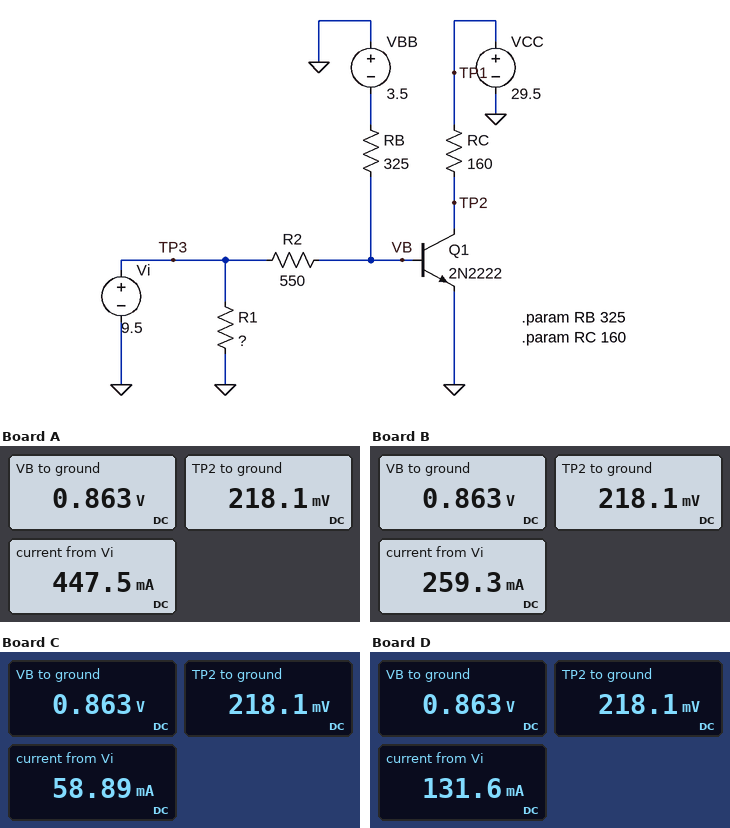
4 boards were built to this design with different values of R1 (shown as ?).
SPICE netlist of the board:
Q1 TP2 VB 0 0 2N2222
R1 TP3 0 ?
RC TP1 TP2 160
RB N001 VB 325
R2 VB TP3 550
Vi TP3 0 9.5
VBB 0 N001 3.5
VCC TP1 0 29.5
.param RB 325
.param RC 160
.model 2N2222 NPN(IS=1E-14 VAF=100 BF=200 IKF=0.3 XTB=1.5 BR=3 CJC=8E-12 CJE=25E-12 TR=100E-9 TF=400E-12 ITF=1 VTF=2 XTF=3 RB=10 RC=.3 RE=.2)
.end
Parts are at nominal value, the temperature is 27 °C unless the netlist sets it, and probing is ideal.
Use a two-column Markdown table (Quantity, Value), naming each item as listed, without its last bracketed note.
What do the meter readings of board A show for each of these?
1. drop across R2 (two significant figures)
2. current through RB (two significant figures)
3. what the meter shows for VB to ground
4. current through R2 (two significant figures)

| Quantity | Value |
|---|---|
| drop across R2 | 8.6 V |
| current through RB | 13 mA |
| what the meter shows for VB to ground | 0.863 V |
| current through R2 | 16 mA |
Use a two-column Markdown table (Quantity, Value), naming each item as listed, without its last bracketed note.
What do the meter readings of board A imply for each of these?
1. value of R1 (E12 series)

| Quantity | Value |
|---|---|
| value of R1 | 22 Ω |
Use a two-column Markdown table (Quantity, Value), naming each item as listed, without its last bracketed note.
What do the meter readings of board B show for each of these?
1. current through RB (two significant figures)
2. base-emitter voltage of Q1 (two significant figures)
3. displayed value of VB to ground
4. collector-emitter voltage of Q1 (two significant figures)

| Quantity | Value |
|---|---|
| current through RB | 13 mA |
| base-emitter voltage of Q1 | 860 mV |
| displayed value of VB to ground | 0.863 V |
| collector-emitter voltage of Q1 | 220 mV |
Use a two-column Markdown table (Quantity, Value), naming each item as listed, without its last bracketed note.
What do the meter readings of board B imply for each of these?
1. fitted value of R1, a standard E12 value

| Quantity | Value |
|---|---|
| fitted value of R1, a standard E12 value | 39 Ω |
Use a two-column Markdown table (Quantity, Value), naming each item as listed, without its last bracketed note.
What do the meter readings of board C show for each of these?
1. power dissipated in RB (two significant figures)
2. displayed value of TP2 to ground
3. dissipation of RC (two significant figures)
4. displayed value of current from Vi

| Quantity | Value |
|---|---|
| power dissipated in RB | 59 mW |
| displayed value of TP2 to ground | 218.1 mV |
| dissipation of RC | 5.4 W |
| displayed value of current from Vi | 58.89 mA |
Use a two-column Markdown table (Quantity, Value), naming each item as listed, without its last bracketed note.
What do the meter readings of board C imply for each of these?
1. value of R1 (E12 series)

| Quantity | Value |
|---|---|
| value of R1 | 220 Ω |
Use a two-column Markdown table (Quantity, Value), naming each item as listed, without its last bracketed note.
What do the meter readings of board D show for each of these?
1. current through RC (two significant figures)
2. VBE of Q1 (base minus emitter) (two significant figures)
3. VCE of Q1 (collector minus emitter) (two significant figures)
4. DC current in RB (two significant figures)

| Quantity | Value |
|---|---|
| current through RC | 180 mA |
| VBE of Q1 (base minus emitter) | 860 mV |
| VCE of Q1 (collector minus emitter) | 220 mV |
| DC current in RB | 13 mA |
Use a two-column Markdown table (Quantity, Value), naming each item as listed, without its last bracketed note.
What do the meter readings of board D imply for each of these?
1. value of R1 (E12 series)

| Quantity | Value |
|---|---|
| value of R1 | 82 Ω |
